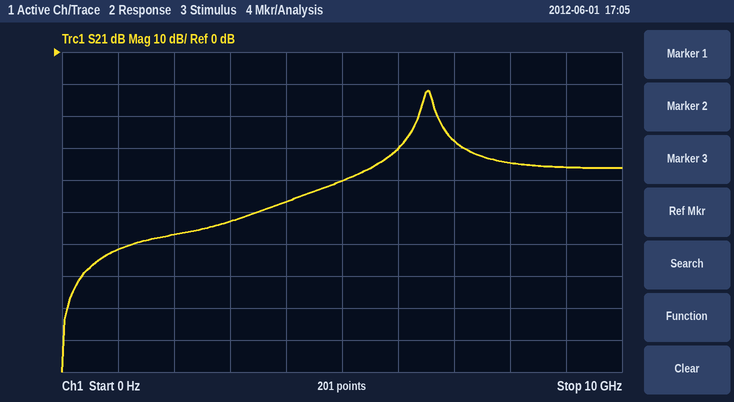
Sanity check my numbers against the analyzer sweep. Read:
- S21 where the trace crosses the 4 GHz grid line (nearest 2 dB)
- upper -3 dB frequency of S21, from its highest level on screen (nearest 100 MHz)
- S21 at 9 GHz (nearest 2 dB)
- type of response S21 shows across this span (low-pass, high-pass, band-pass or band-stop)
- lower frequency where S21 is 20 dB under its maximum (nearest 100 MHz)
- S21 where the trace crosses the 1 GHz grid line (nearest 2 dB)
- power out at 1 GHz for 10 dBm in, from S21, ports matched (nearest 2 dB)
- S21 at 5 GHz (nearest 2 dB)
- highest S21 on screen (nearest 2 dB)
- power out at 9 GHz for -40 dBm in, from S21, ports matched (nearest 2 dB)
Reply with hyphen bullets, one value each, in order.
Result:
- -46 dB
- 6.6 GHz
- -36 dB
- band-pass
- 5.9 GHz
- -62 dB
- -52 dBm
- -40 dB
- -12 dB
- -76 dBm
